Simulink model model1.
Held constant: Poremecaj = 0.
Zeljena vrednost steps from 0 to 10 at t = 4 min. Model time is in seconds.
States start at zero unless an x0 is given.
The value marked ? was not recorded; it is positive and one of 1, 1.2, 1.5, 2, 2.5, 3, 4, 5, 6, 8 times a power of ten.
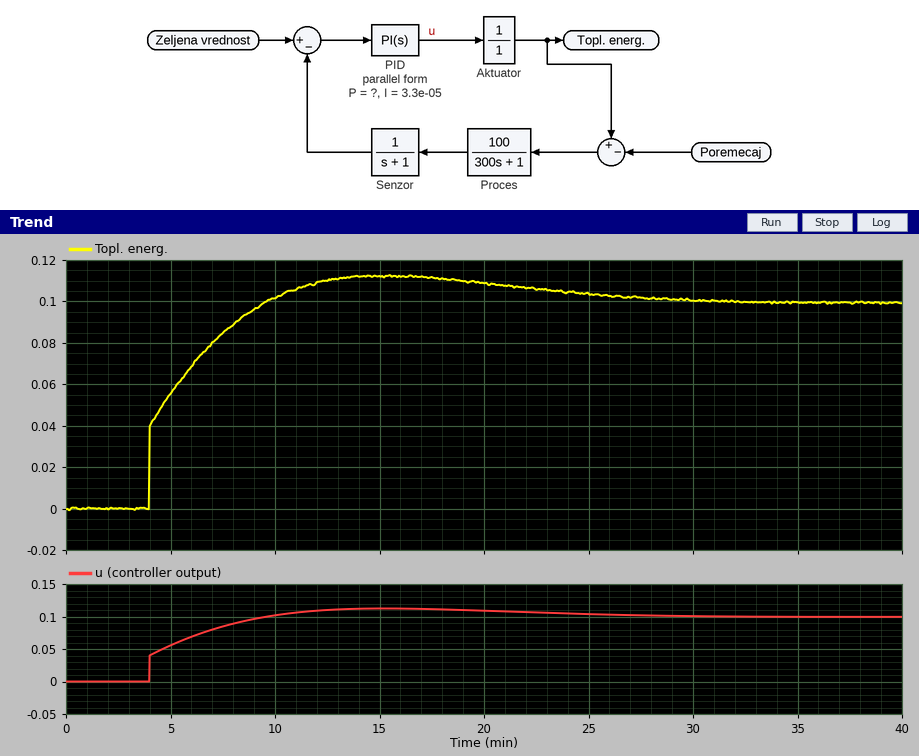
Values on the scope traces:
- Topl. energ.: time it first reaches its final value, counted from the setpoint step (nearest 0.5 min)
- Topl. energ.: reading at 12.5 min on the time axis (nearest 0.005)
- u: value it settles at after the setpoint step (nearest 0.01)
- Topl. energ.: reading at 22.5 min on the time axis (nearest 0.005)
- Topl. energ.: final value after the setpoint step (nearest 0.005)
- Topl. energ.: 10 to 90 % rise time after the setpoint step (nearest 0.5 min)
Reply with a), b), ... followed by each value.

a) 5.5 min
b) 0.110
c) 0.10
d) 0.105
e) 0.100
f) 4.0 min
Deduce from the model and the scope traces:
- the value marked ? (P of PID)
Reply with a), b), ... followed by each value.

a) 0.004
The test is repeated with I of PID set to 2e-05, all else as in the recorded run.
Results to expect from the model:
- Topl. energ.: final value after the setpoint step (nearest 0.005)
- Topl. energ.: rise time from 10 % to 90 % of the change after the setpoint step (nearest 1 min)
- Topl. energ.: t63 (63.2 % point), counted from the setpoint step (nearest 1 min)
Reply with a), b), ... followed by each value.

a) 0.100
b) 10 min
c) 3 min
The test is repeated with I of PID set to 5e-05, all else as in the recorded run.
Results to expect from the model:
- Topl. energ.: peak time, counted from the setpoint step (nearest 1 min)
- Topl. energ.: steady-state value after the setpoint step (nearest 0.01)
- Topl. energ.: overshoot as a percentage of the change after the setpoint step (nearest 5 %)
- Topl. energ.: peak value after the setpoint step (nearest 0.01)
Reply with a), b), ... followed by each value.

a) 8 min
b) 0.10
c) 30 %
d) 0.13
